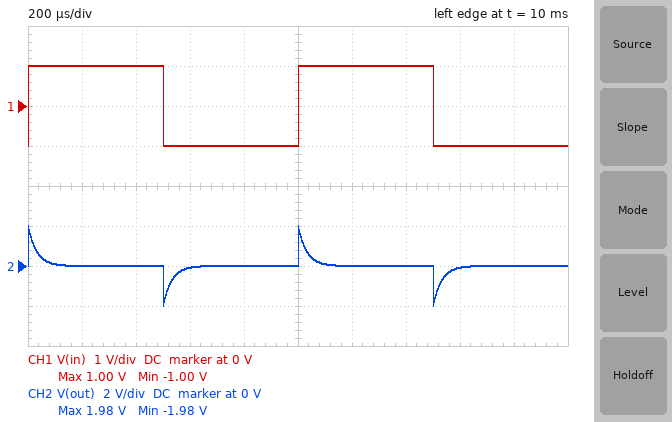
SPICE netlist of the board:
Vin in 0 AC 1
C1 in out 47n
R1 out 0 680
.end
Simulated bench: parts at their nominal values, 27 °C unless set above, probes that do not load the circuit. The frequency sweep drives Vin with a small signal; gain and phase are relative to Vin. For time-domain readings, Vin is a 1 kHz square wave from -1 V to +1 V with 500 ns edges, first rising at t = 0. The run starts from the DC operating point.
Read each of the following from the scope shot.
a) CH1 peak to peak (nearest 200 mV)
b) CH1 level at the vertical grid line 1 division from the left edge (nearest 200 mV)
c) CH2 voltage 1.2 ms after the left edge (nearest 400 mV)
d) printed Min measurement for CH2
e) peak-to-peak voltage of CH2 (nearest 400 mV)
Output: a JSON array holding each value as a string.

["2.0 V", "1.0 V", "0 V", "-1.98 V", "4.0 V"]
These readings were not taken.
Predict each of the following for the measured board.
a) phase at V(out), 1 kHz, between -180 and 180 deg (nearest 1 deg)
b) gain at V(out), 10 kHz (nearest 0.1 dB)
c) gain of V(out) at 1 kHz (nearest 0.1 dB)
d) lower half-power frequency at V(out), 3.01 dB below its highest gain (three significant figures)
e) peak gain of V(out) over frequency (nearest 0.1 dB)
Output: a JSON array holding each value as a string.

["79 deg", "-1.0 dB", "-14.1 dB", "4.98 kHz", "0 dB"]
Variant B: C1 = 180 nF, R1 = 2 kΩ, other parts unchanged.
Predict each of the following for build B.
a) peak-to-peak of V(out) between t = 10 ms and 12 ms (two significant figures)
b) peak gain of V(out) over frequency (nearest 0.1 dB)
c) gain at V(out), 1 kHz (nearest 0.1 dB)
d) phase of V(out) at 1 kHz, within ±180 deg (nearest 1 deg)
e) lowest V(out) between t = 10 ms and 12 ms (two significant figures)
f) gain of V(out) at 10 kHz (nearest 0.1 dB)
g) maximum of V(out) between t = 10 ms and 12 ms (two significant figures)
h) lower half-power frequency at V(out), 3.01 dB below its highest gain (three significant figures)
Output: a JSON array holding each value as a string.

["3.2 V", "0 dB", "-0.8 dB", "24 deg", "-1.6 V", "0 dB", "1.6 V", "442 Hz"]
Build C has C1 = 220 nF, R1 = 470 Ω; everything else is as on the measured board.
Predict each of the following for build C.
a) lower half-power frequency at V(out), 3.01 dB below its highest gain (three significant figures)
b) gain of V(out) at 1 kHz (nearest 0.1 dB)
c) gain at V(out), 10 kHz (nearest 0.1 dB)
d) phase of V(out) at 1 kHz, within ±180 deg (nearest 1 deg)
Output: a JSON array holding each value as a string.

["1.54 kHz", "-5.3 dB", "-0.1 dB", "57 deg"]
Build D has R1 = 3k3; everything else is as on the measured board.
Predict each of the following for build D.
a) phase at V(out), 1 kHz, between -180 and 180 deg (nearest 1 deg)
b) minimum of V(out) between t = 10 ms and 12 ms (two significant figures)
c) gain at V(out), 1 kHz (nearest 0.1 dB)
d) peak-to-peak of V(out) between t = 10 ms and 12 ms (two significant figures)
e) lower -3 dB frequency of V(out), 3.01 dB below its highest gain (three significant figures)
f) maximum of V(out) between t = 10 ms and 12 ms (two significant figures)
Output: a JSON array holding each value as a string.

["46 deg", "-1.9 V", "-3.1 dB", "3.8 V", "1.03 kHz", "1.9 V"]
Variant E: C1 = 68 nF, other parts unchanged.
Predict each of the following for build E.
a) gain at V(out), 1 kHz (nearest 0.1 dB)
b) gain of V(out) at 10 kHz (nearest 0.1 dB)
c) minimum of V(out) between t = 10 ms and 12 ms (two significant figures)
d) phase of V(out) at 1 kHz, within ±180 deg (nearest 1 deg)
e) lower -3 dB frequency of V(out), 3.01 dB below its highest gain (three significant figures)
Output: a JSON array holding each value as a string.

["-11.1 dB", "-0.5 dB", "-2.0 V", "74 deg", "3.44 kHz"]
